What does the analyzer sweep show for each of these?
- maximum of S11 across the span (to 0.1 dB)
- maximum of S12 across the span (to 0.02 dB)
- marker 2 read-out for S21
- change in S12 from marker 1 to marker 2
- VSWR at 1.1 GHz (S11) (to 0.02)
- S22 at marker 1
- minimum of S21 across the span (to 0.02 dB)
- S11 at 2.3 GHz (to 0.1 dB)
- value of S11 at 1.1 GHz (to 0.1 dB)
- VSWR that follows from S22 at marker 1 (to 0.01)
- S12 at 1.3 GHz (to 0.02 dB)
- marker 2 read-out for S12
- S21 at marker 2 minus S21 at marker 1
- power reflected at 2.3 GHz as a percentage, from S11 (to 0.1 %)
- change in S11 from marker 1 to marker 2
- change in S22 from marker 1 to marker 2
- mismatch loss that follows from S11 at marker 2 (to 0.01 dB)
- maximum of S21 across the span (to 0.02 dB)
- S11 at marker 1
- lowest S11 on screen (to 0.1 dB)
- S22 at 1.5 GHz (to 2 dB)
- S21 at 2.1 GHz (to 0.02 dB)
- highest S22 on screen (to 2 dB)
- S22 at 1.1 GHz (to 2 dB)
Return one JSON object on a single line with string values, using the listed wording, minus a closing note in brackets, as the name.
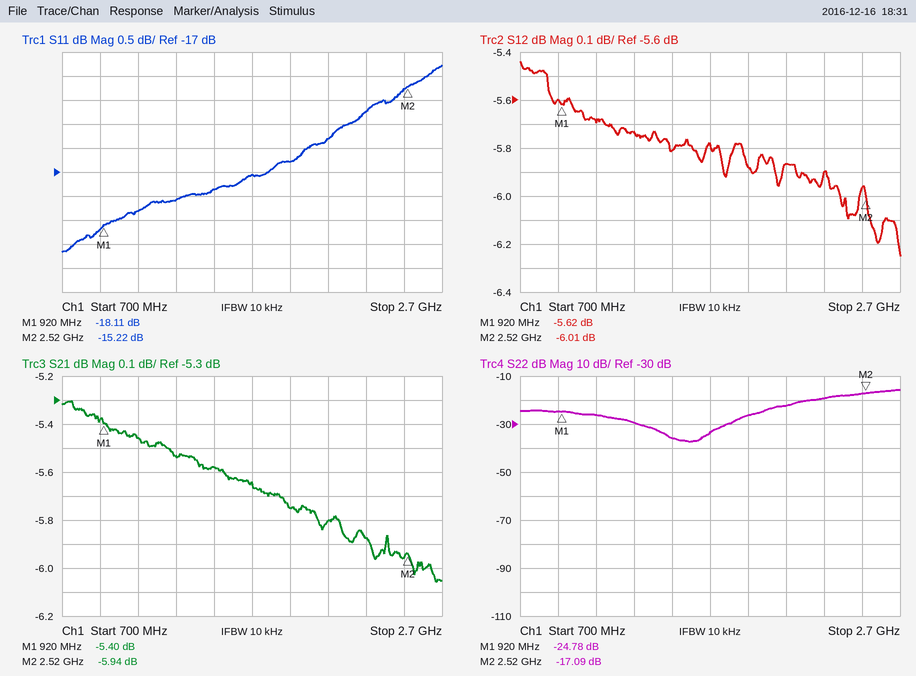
{"maximum of S11 across the span": "-14.8 dB", "maximum of S12 across the span": "-5.44 dB", "marker 2 read-out for S21": "-5.94 dB", "change in S12 from marker 1 to marker 2": "-0.39 dB", "VSWR at 1.1 GHz (S11)": "1.30", "S22 at marker 1": "-24.78 dB", "minimum of S21 across the span": "-6.06 dB", "S11 at 2.3 GHz": "-15.7 dB", "value of S11 at 1.1 GHz": "-17.8 dB", "VSWR that follows from S22 at marker 1": "1.12", "S12 at 1.3 GHz": "-5.74 dB", "marker 2 read-out for S12": "-6.01 dB", "S21 at marker 2 minus S21 at marker 1": "-0.54 dB", "power reflected at 2.3 GHz as a percentage, from S11": "2.7 %", "change in S11 from marker 1 to marker 2": "2.89 dB", "change in S22 from marker 1 to marker 2": "7.69 dB", "mismatch loss that follows from S11 at marker 2": "0.13 dB", "maximum of S21 across the span": "-5.30 dB", "S11 at marker 1": "-18.11 dB", "lowest S11 on screen": "-18.7 dB", "S22 at 1.5 GHz": "-36 dB", "S21 at 2.1 GHz": "-5.80 dB", "highest S22 on screen": "-16 dB", "S22 at 1.1 GHz": "-26 dB"}
